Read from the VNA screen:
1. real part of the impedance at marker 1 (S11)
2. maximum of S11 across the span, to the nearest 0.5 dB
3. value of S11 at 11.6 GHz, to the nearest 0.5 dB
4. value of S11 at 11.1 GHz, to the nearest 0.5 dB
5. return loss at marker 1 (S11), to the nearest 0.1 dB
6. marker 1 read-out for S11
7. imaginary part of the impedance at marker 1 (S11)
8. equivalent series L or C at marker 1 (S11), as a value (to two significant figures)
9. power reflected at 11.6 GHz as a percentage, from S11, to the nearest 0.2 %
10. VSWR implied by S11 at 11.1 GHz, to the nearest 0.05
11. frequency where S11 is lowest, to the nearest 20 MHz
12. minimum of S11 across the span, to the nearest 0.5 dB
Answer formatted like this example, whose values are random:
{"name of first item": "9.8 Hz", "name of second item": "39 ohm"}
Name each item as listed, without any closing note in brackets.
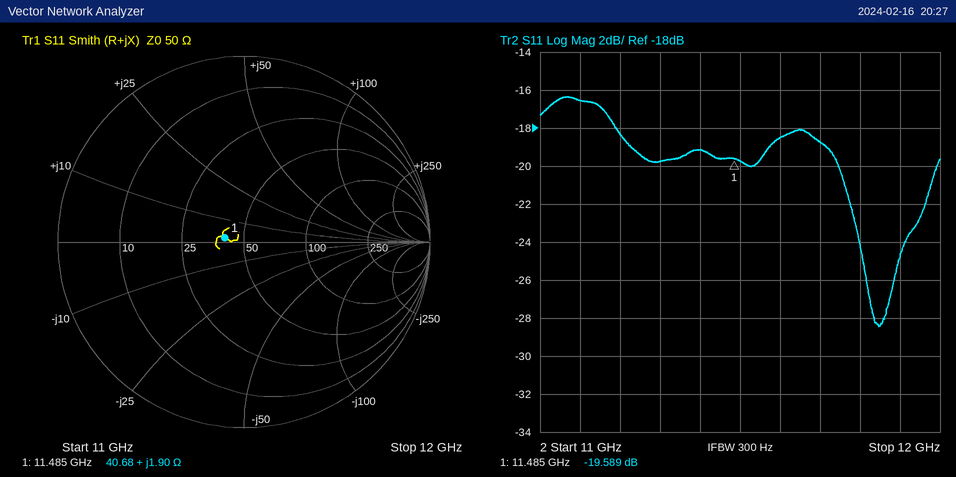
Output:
{"real part of the impedance at marker 1": "40.68 Ω", "maximum of S11 across the span, to the nearest 0.5 dB": "-16.5 dB", "value of S11 at 11.6 GHz, to the nearest 0.5 dB": "-18.5 dB", "value of S11 at 11.1 GHz, to the nearest 0.5 dB": "-16.5 dB", "return loss at marker 1 (S11), to the nearest 0.1 dB": "19.6 dB", "marker 1 read-out for S11": "-19.589 dB", "imaginary part of the impedance at marker 1": "+1.90 Ω", "equivalent series L or C at marker 1 (S11), as a value": "26 pH", "power reflected at 11.6 GHz as a percentage, from S11, to the nearest 0.2 %": "1.4 %", "VSWR implied by S11 at 11.1 GHz, to the nearest 0.05": "1.35", "frequency where S11 is lowest, to the nearest 20 MHz": "11.84 GHz", "minimum of S11 across the span, to the nearest 0.5 dB": "-28.5 dB"}
